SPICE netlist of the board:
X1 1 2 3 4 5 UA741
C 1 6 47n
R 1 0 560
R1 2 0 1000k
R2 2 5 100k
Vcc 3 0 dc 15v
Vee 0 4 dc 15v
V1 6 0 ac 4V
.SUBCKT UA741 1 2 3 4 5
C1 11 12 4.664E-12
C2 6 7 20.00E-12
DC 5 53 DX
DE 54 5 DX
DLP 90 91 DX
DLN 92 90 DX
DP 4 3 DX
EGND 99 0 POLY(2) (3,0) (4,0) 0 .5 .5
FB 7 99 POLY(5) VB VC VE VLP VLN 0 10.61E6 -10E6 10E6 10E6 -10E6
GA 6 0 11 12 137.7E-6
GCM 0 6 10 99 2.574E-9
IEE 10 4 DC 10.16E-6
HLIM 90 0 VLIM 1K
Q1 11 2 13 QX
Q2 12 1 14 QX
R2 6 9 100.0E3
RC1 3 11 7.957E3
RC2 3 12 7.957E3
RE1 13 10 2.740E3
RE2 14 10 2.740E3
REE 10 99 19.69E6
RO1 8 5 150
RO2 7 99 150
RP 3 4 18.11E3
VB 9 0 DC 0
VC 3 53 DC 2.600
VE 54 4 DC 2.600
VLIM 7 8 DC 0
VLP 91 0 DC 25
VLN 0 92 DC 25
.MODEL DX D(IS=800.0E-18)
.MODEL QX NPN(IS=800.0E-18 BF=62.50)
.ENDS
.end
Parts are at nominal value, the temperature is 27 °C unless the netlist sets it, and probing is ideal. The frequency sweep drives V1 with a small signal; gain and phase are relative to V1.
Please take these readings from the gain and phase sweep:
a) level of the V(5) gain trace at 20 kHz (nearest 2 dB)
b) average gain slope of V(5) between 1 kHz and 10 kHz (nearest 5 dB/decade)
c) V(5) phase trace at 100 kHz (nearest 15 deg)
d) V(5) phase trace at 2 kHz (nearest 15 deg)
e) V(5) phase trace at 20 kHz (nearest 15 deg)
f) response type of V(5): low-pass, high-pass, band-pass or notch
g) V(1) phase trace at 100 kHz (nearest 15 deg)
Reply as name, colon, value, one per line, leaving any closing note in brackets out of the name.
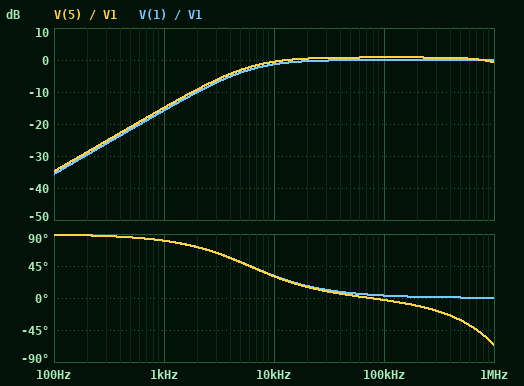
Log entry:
level of the V(5) gain trace at 20 kHz: 0 dB
average gain slope of V(5) between 1 kHz and 10 kHz: 15 dB/decade
V(5) phase trace at 100 kHz: 0 deg
V(5) phase trace at 2 kHz: 75 deg
V(5) phase trace at 20 kHz: 15 deg
response type of V(5): low-pass, high-pass, band-pass or notch: high-pass
V(1) phase trace at 100 kHz: 0 deg
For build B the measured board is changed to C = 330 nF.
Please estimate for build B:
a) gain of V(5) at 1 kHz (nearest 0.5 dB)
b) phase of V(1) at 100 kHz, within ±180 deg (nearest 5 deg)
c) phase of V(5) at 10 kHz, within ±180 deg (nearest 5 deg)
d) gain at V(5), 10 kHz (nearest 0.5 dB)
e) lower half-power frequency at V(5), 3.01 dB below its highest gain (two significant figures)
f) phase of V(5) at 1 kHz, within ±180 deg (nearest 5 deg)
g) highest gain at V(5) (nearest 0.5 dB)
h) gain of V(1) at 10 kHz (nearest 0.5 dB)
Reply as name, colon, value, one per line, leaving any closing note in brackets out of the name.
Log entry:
gain of V(5) at 1 kHz: -1.5 dB
phase of V(1) at 100 kHz, within ±180 deg: 0 deg
phase of V(5) at 10 kHz, within ±180 deg: 5 deg
gain at V(5), 10 kHz: 1.0 dB
lower half-power frequency at V(5), 3.01 dB below its highest gain: 860 Hz
phase of V(5) at 1 kHz, within ±180 deg: 40 deg
highest gain at V(5): 1.0 dB
gain of V(1) at 10 kHz: 0 dB
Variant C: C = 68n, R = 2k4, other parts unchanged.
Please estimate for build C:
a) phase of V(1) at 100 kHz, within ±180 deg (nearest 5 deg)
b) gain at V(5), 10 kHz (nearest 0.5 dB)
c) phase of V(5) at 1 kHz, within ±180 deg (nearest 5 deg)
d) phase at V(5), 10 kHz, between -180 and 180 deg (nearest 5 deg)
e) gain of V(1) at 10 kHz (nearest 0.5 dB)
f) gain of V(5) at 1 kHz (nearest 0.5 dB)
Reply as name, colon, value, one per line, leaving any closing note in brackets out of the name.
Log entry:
phase of V(1) at 100 kHz, within ±180 deg: 0 deg
gain at V(5), 10 kHz: 1.0 dB
phase of V(5) at 1 kHz, within ±180 deg: 45 deg
phase at V(5), 10 kHz, between -180 and 180 deg: 5 deg
gain of V(1) at 10 kHz: 0 dB
gain of V(5) at 1 kHz: -2.0 dB
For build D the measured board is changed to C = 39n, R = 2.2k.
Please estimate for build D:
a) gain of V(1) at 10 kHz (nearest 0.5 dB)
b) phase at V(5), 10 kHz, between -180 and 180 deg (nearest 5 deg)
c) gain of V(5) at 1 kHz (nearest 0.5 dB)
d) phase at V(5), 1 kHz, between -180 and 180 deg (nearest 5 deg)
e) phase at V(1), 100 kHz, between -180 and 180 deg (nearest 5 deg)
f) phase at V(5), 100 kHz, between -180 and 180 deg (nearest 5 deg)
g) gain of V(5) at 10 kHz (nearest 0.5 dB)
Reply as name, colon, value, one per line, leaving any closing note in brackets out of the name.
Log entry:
gain of V(1) at 10 kHz: 0 dB
phase at V(5), 10 kHz, between -180 and 180 deg: 10 deg
gain of V(5) at 1 kHz: -5.5 dB
phase at V(5), 1 kHz, between -180 and 180 deg: 60 deg
phase at V(1), 100 kHz, between -180 and 180 deg: 0 deg
phase at V(5), 100 kHz, between -180 and 180 deg: -5 deg
gain of V(5) at 10 kHz: 0.5 dB
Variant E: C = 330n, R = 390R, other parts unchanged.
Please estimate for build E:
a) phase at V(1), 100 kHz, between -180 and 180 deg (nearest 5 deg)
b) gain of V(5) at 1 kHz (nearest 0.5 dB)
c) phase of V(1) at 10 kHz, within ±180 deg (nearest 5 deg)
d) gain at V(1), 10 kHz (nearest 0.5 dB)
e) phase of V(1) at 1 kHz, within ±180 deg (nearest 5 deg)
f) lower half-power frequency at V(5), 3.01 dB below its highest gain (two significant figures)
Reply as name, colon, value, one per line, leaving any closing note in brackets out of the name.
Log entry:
phase at V(1), 100 kHz, between -180 and 180 deg: 0 deg
gain of V(5) at 1 kHz: -3.0 dB
phase of V(1) at 10 kHz, within ±180 deg: 5 deg
gain at V(1), 10 kHz: 0 dB
phase of V(1) at 1 kHz, within ±180 deg: 50 deg
lower half-power frequency at V(5), 3.01 dB below its highest gain: 1.2 kHz
